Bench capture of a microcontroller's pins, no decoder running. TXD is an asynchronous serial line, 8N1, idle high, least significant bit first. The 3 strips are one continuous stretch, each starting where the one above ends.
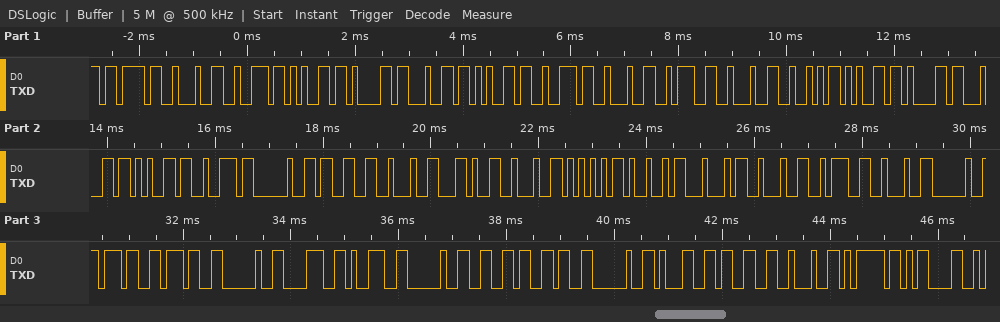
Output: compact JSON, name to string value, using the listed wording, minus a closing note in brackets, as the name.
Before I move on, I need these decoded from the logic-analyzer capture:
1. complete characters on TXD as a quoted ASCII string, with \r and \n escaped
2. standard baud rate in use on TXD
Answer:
{"complete characters on TXD as a quoted ASCII string, with \\r and \\n escaped": "\"{\\\"reader\\\":\\\"Reader 3\\\",\\\"UID\\\":\\\" 77 89 f6 13\\\"}\\r\"", "standard baud rate in use on TXD": "9600 baud"}
